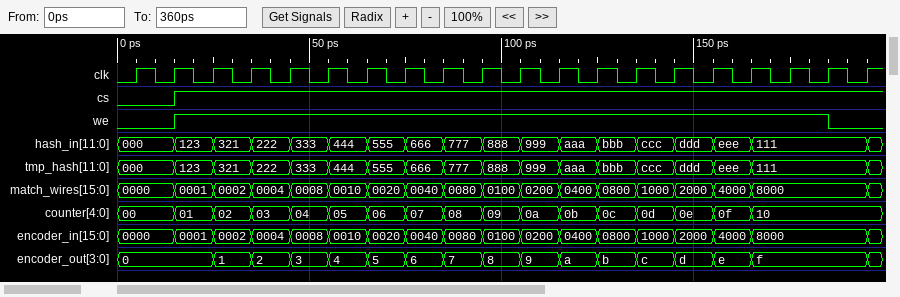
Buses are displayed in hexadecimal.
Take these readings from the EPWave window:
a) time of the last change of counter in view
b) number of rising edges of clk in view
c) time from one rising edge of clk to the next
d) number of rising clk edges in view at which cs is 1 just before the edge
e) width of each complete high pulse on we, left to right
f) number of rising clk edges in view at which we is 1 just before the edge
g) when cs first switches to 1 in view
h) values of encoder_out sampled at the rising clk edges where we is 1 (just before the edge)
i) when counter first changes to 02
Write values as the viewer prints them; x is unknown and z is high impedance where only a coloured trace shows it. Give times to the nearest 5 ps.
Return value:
165 ps
20
10 ps
18
170 ps
17
15 ps
0, 1, 2, 3, 4, 5, 6, 7, 8, 9, a, b, c, d, e, f, f
25 ps
